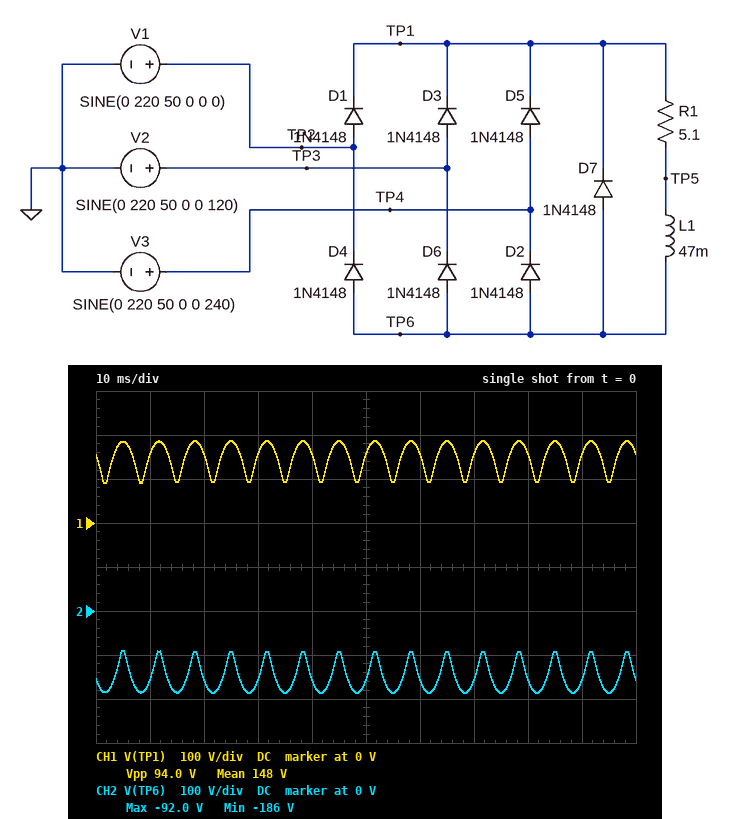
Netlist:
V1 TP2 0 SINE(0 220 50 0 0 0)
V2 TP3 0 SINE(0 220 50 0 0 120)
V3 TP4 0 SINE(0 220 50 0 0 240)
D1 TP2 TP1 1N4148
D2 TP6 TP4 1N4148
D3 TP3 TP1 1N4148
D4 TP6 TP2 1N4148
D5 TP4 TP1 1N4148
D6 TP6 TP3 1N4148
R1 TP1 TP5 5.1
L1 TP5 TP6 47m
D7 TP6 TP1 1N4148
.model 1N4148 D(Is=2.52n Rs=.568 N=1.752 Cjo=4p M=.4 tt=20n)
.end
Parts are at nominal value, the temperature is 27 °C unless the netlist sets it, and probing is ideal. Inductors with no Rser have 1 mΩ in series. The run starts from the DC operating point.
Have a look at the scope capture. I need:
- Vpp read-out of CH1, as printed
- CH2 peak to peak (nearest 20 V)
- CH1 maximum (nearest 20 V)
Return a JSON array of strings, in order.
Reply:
["94.0 V", "100 V", "180 V"]
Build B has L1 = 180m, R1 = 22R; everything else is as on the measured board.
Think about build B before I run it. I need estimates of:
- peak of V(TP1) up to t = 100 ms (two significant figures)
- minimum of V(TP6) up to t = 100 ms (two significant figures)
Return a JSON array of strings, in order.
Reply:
["210 V", "-210 V"]
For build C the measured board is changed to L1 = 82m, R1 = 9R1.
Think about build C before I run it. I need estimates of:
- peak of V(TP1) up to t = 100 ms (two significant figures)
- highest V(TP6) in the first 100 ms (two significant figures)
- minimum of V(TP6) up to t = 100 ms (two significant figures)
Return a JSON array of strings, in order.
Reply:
["200 V", "-99 V", "-200 V"]
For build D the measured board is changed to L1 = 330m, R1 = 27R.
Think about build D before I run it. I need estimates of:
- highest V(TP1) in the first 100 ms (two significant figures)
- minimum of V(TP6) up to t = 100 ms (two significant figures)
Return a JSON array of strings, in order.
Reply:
["210 V", "-210 V"]
